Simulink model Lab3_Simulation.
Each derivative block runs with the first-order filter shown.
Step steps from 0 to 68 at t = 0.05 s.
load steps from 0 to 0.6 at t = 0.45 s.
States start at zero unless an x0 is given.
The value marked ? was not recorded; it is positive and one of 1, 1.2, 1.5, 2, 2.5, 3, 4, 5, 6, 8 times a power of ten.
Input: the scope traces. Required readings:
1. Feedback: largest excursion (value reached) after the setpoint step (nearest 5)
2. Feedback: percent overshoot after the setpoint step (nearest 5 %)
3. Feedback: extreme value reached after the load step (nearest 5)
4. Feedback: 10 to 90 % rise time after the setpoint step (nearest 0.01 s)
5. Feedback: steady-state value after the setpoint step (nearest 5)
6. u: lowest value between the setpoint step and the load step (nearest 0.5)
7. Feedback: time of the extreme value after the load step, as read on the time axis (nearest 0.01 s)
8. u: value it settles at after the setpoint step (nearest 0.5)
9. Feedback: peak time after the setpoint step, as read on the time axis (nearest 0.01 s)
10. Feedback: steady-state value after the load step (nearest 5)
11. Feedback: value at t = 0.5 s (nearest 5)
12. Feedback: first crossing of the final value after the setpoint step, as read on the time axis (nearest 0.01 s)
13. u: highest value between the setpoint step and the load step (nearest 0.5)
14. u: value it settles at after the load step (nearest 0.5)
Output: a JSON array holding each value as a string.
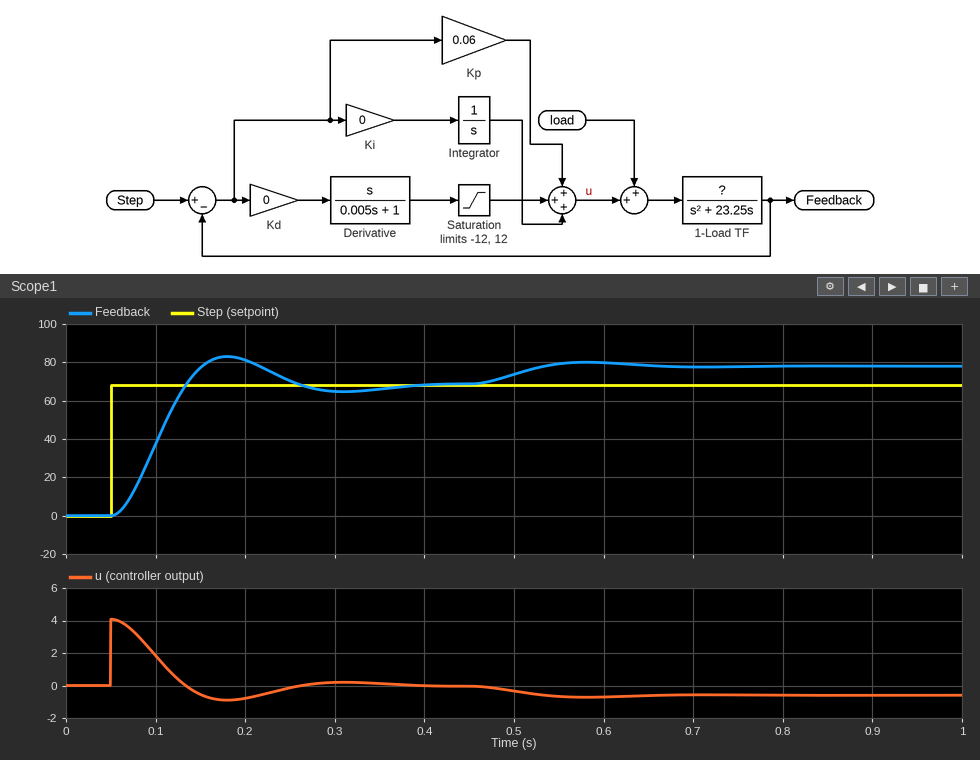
["85", "20 %", "80", "0.06 s", "70", "-1.0", "0.58 s", "0.0", "0.18 s", "80", "75", "0.13 s", "4.0", "-0.5"]
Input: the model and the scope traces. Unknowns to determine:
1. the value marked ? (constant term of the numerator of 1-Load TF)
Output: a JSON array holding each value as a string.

["12000"]
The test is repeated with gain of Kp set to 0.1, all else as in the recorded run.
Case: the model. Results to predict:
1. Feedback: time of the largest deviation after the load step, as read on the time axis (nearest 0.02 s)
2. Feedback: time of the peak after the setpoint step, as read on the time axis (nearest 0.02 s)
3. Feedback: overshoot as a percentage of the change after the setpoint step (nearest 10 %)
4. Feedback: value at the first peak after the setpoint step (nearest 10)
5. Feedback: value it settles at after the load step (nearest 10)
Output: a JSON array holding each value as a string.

["0.54 s", "0.14 s", "30 %", "90", "70"]
